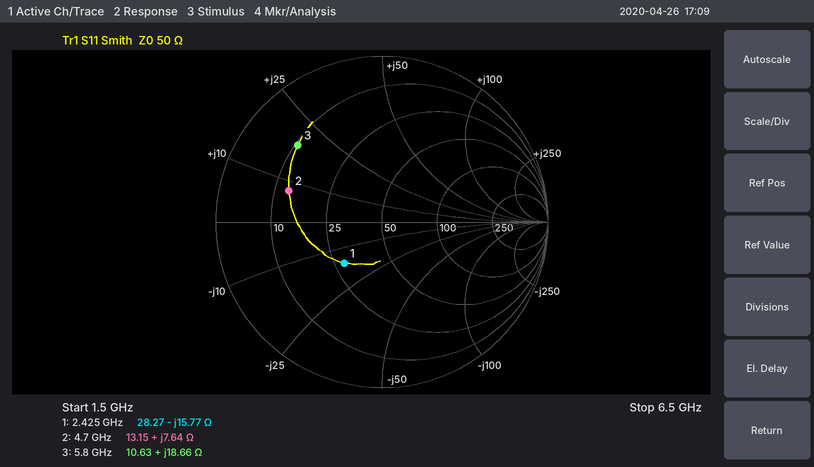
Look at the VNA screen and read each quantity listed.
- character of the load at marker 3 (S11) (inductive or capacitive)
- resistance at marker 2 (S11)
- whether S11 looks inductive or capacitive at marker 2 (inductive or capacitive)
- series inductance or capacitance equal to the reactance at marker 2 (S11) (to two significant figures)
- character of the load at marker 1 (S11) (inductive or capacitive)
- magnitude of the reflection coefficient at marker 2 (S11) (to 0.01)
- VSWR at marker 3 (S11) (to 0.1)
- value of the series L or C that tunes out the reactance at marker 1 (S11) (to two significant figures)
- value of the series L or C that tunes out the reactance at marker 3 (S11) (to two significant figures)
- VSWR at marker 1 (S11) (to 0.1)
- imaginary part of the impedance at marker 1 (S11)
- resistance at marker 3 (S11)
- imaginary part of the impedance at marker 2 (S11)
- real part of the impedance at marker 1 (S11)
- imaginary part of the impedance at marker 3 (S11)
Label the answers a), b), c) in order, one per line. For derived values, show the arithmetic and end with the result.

a) inductive
b) 13.15 Ω
c) inductive
d) L = 7.64 Ω/(2π × 4.7 GHz) ≈ 259 pH, so 260 pH to two significant figures
e) capacitive
f) 0.59
g) 5.4
h) L = 15.77 Ω/(2π × 2.425 GHz) ≈ 1.0 nH
i) C = 1/(2π × 5.8 GHz × 18.66 Ω) ≈ 1.5 pF
j) 2.0
k) -15.77 Ω
l) 10.63 Ω
m) +7.64 Ω
n) 28.27 Ω
o) +18.66 Ω
